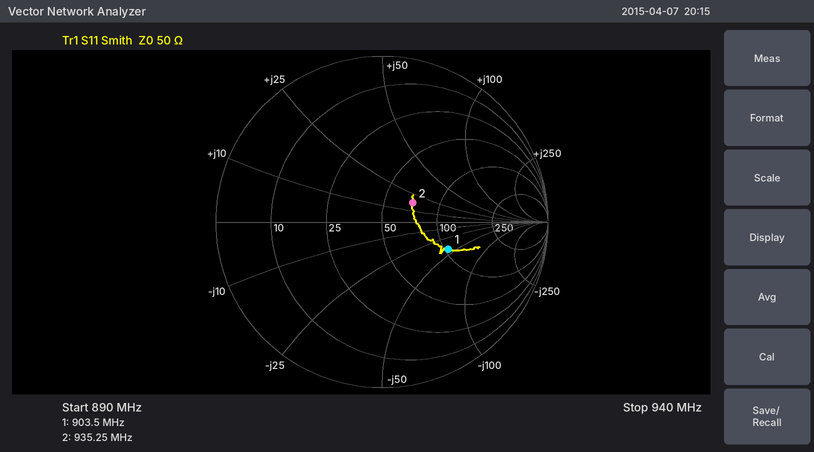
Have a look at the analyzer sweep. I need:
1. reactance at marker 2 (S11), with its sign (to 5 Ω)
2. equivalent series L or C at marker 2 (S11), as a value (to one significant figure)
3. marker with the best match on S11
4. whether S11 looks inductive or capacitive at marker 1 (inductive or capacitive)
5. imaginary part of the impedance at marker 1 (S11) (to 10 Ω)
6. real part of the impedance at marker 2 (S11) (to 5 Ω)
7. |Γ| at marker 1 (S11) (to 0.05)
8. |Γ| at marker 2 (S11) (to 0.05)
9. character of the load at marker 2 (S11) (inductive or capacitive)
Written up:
+15 Ω
3 nH
marker 2
capacitive
-40 Ω
70 Ω
0.45
0.20
inductive
